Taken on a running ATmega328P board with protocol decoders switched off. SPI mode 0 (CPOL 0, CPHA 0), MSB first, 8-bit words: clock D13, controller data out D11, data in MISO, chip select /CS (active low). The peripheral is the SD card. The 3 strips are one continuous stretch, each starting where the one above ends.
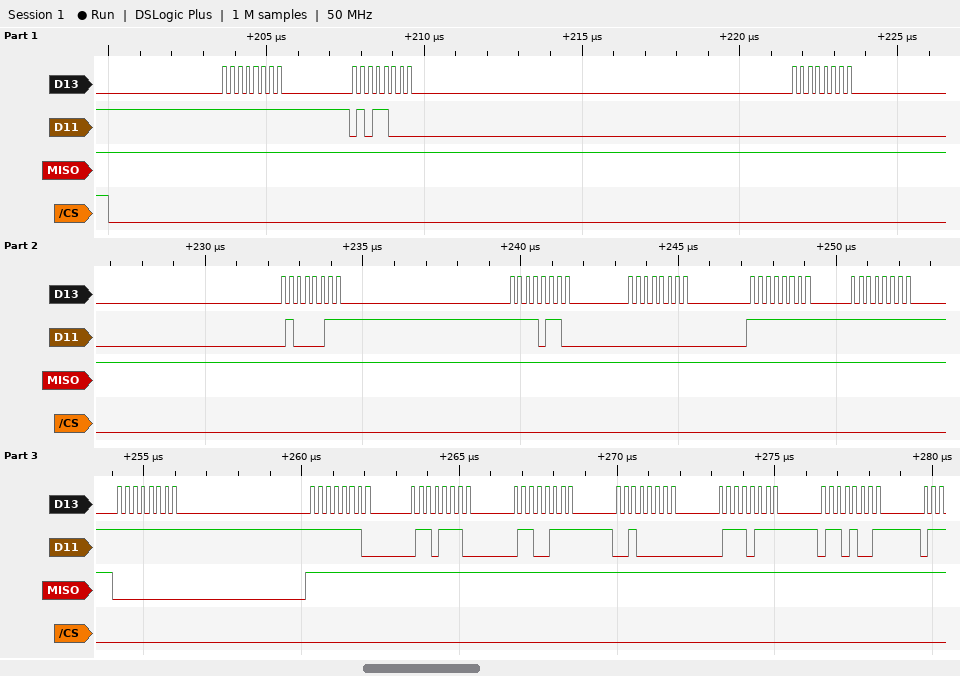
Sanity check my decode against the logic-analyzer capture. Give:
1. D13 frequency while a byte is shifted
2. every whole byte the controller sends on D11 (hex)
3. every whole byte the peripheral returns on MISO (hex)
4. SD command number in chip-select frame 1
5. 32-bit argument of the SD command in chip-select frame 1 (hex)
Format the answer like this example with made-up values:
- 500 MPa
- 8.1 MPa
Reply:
- 4 MHz
- 0xFF 0x58 0x00 0x43 0xF6 0x00 0xFF 0xFF 0xFF 0xFE 0x6E 0x67 0x20 0x77 0x69
- 0xFF 0xFF 0xFF 0xFF 0xFF 0xFF 0xFF 0xFF 0x00 0xFF 0xFF 0xFF 0xFF 0xFF 0xFF
- CMD24
- 0x0043F600
